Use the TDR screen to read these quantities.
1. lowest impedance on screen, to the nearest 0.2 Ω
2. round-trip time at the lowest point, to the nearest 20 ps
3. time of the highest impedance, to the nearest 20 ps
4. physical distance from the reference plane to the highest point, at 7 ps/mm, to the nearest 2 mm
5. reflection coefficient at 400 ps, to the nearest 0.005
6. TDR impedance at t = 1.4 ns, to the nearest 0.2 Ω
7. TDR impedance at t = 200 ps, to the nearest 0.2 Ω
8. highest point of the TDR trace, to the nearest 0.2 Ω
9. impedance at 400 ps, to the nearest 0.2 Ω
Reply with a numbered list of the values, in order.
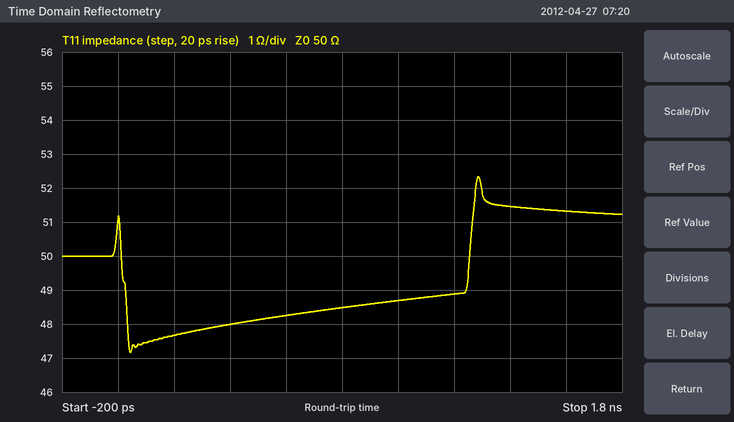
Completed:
1. 47.2 Ω
2. 40 ps
3. 1.28 ns
4. 92 mm
5. -0.020
6. 51.4 Ω
7. 47.6 Ω
8. 52.4 Ω
9. 48.0 Ω
